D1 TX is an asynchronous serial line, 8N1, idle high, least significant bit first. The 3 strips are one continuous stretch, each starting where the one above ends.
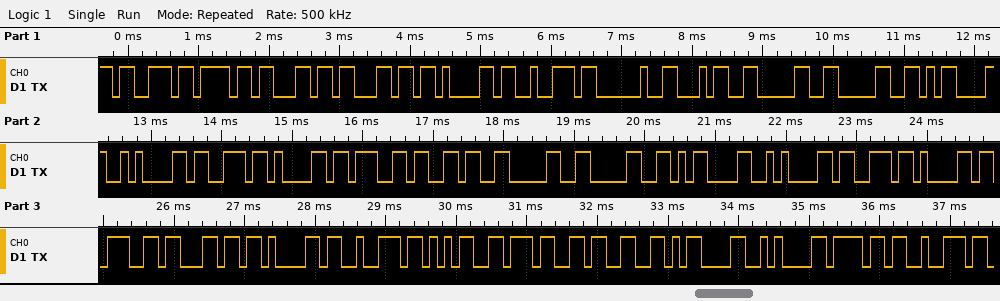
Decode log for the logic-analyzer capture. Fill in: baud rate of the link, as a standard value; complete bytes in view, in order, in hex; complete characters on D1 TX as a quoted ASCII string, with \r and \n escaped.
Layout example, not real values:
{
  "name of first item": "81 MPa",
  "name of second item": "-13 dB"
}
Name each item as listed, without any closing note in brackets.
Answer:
{
  "baud rate of the link, as a standard value": "9600 baud",
  "complete bytes in view, in order, in hex": "0x73 0x6F 0x6C 0x6C 0x61 0x72 0x20 0x34 0x30 0x30 0x0D 0x0A 0x73 0x61 0x67 0x36 0x30 0x30 0x0D 0x0A 0x73 0x61 0x67 0x6C 0x61 0x72 0x35 0x37 0x33 0x0D 0x0A 0x6F 0x72",
  "complete characters on D1 TX as a quoted ASCII string, with \\r and \\n escaped": "\"sollar 400\\r\\nsag600\\r\\nsaglar573\\r\\nor\""
}
